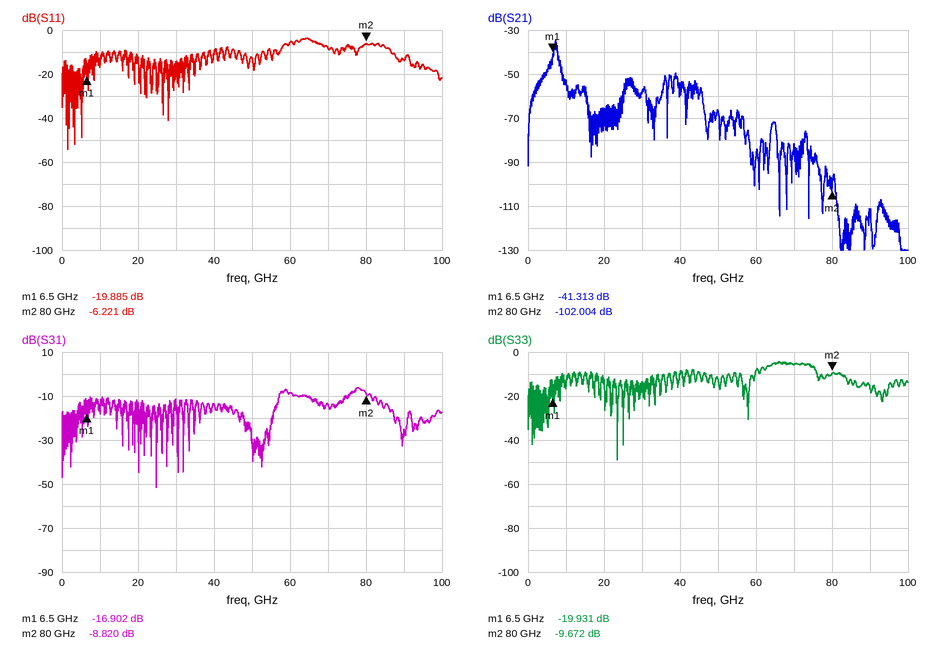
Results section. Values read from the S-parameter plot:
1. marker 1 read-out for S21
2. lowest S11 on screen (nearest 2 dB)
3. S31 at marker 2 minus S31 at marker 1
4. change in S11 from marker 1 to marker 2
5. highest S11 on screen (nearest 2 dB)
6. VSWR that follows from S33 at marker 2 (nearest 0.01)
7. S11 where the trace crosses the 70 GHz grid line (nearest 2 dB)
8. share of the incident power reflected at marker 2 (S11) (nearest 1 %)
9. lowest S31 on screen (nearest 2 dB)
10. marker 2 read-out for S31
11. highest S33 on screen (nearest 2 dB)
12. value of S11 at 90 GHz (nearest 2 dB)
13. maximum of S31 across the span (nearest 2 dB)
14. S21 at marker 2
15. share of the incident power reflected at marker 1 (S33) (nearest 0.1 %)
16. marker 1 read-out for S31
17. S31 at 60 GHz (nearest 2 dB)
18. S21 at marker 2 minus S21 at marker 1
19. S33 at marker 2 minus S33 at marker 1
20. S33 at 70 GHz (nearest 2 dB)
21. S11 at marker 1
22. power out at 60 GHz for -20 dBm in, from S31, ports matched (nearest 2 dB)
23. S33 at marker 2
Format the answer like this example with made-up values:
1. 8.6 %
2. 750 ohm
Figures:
1. -41.313 dB
2. -54 dB
3. 8.082 dB
4. 13.664 dB
5. -4 dB
6. 1.98
7. -8 dB
8. 24 %
9. -52 dB
10. -8.820 dB
11. -4 dB
12. -14 dB
13. -6 dB
14. -102.004 dB
15. 1.0 %
16. -16.902 dB
17. -8 dB
18. -60.691 dB
19. 10.259 dB
20. -6 dB
21. -19.885 dB
22. -28 dBm
23. -9.672 dB
